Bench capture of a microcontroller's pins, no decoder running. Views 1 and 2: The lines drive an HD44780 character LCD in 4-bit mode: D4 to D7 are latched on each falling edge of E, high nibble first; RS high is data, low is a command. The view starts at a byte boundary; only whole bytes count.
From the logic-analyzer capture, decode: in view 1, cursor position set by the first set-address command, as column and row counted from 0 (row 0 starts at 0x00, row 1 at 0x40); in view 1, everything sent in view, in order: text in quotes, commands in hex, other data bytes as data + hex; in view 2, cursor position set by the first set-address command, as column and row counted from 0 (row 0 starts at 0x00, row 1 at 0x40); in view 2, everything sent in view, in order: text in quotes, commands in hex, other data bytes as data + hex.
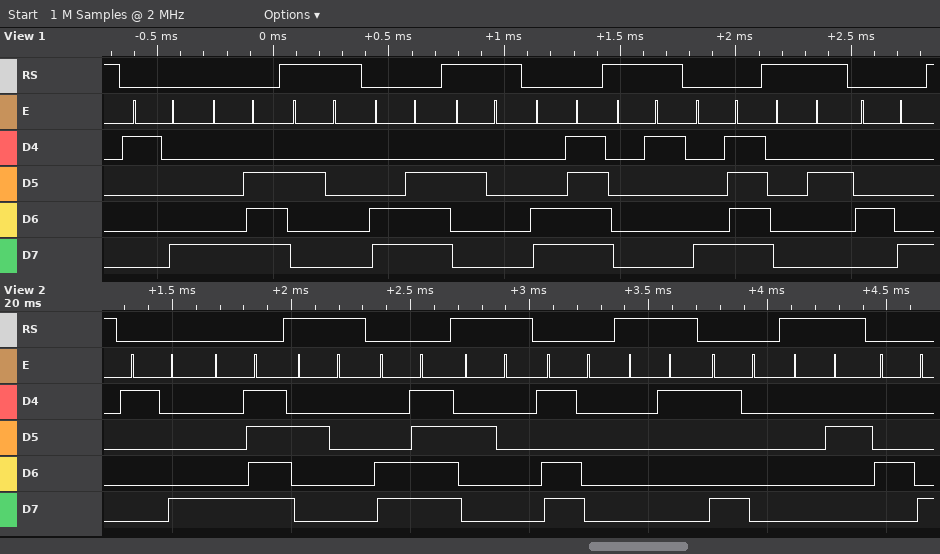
column 14, row 0
0x18 0x8E " " 0xCE " " 0xCF data 01 0x8F data 02 0x48
column 15, row 0
0x18 0x8F " " 0xCF " " 0xD0 data 01 0x90 data 02 0x48
